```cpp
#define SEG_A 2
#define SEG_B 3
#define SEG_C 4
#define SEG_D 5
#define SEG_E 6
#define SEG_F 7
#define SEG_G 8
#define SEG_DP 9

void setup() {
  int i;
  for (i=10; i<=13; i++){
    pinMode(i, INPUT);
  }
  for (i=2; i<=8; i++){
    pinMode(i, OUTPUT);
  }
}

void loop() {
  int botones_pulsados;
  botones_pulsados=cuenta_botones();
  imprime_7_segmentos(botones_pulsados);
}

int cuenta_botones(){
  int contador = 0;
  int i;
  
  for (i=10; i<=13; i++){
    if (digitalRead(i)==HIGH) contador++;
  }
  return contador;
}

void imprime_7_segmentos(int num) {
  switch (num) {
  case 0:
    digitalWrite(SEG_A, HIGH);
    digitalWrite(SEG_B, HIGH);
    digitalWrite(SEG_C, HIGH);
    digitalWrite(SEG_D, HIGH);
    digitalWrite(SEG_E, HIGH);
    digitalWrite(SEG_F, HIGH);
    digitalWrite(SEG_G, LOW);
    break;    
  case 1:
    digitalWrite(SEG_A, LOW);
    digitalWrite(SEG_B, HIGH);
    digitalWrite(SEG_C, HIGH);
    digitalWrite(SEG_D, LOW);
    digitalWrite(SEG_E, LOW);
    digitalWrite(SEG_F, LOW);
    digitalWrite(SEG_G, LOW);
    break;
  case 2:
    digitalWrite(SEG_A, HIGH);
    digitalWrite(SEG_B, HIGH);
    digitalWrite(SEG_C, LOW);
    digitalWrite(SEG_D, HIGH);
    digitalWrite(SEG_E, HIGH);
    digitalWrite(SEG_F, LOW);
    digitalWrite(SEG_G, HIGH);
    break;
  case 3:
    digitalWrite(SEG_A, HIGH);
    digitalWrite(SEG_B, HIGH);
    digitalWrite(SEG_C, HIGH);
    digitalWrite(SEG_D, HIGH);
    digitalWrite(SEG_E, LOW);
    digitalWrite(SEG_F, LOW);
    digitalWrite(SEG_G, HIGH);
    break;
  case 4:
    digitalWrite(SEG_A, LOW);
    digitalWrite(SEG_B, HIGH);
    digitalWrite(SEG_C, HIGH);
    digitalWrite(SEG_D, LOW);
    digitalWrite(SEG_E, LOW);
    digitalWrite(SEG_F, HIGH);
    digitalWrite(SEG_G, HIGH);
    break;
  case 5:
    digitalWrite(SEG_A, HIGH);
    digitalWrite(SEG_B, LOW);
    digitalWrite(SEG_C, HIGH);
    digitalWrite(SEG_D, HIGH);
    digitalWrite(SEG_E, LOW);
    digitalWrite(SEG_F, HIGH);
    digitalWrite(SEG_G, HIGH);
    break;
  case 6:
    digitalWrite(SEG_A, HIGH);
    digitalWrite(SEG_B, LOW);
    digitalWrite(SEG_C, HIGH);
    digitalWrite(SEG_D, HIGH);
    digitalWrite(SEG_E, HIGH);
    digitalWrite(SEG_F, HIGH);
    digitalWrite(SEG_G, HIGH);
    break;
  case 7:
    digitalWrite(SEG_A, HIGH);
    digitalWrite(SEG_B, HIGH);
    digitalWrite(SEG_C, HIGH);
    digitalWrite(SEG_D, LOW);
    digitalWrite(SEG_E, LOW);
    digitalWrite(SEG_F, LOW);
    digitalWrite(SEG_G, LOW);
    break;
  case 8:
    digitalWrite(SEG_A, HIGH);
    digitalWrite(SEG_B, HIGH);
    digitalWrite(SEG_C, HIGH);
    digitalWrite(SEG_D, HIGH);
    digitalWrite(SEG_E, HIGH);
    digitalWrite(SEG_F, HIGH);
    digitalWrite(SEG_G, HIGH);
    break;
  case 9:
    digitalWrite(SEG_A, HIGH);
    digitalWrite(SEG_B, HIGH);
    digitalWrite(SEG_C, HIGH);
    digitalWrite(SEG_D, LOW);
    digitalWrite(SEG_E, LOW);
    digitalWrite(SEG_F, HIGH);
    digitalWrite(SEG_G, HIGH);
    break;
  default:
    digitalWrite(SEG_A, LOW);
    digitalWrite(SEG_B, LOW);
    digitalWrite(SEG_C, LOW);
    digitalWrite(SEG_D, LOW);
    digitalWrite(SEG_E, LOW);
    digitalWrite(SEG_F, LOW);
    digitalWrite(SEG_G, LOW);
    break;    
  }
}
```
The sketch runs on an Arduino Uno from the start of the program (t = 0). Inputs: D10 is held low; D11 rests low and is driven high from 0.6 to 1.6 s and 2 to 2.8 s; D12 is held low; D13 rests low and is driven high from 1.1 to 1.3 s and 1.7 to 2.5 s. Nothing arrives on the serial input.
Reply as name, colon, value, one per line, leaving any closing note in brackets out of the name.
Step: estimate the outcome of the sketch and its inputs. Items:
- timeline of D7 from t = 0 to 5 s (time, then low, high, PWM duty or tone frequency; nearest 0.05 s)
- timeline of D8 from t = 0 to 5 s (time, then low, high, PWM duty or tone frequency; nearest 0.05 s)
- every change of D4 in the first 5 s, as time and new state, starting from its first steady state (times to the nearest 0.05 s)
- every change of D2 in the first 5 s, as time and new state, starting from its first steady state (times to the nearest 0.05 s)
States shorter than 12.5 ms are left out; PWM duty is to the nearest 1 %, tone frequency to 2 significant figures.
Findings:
timeline of D7 from t = 0 to 5 s: 0 s high; 0.6 s low; 1.6 s high; 1.7 s low; 2.8 s high
timeline of D8 from t = 0 to 5 s: 0 s low; 1.1 s high; 1.3 s low; 2 s high; 2.5 s low
every change of D4 in the first 5 s, as time and new state, starting from its first steady state: 0 s high; 1.1 s low; 1.3 s high; 2 s low; 2.5 s high
every change of D2 in the first 5 s, as time and new state, starting from its first steady state: 0 s high; 0.6 s low; 1.1 s high; 1.3 s low; 1.6 s high; 1.7 s low; 2 s high; 2.5 s low; 2.8 s high
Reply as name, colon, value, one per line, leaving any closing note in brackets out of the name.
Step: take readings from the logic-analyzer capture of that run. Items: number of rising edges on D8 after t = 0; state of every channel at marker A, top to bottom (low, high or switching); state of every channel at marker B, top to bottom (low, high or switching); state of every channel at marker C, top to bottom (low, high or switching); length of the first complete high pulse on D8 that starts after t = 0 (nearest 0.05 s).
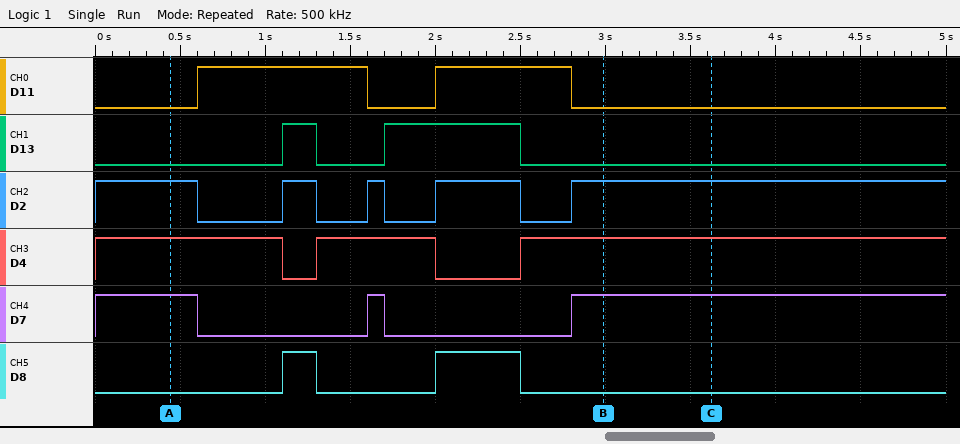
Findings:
number of rising edges on D8 after t = 0: 2
state of every channel at marker A, top to bottom: D11 low, D13 low, D2 high, D4 high, D7 high, D8 low
state of every channel at marker B, top to bottom: D11 low, D13 low, D2 high, D4 high, D7 high, D8 low
state of every channel at marker C, top to bottom: D11 low, D13 low, D2 high, D4 high, D7 high, D8 low
length of the first complete high pulse on D8 that starts after t = 0: 0.20 s
